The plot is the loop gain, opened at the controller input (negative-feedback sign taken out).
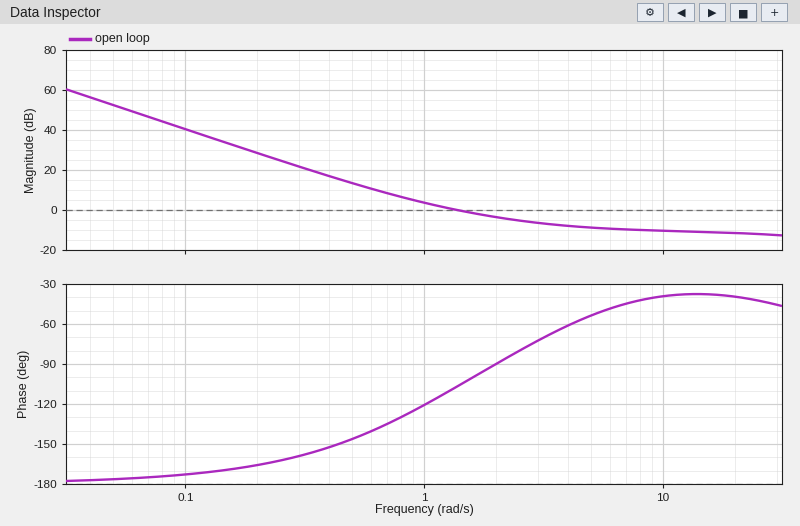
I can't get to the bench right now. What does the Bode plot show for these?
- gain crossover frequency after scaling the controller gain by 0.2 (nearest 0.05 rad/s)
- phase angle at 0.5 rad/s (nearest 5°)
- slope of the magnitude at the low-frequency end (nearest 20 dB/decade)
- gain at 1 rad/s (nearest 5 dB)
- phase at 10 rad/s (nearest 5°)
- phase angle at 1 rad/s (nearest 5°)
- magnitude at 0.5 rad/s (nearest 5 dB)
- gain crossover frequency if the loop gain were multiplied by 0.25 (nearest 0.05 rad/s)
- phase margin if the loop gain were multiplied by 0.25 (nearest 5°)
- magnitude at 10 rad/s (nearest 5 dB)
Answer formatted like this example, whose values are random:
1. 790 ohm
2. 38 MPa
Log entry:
1. 0.50 rad/s
2. -145°
3. -40 dB/decade
4. 5 dB
5. -40°
6. -120°
7. 15 dB
8. 0.55 rad/s
9. 35°
10. -10 dB
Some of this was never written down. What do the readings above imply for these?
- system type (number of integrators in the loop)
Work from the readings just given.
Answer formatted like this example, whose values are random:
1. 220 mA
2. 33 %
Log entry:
1. 2
